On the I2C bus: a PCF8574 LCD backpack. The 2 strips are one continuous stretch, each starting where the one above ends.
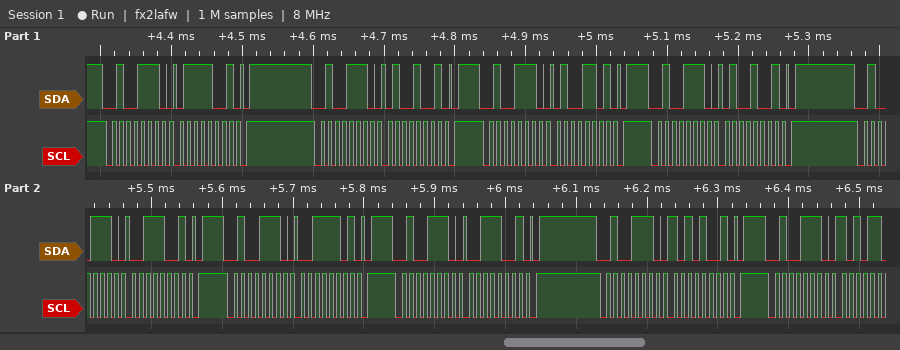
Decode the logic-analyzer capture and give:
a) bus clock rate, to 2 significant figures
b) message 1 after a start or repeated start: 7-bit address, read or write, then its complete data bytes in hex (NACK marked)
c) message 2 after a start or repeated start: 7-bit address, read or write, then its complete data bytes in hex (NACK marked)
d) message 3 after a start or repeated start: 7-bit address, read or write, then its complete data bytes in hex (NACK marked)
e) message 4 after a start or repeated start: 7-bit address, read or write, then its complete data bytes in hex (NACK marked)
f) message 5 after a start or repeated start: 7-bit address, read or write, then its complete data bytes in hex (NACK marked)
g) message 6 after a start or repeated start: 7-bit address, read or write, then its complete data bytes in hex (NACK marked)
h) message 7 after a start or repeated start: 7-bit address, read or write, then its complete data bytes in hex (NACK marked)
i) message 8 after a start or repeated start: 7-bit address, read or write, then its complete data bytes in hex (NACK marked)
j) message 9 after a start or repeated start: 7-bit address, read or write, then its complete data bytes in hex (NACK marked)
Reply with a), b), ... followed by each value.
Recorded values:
a) 100 kHz
b) 0x27 write: 79
c) 0x27 write: 49
d) 0x27 write: 4D
e) 0x27 write: 49
f) 0x27 write: 39
g) 0x27 write: 3D
h) 0x27 write: 39
i) 0x27 write: A9
j) 0x27 write
